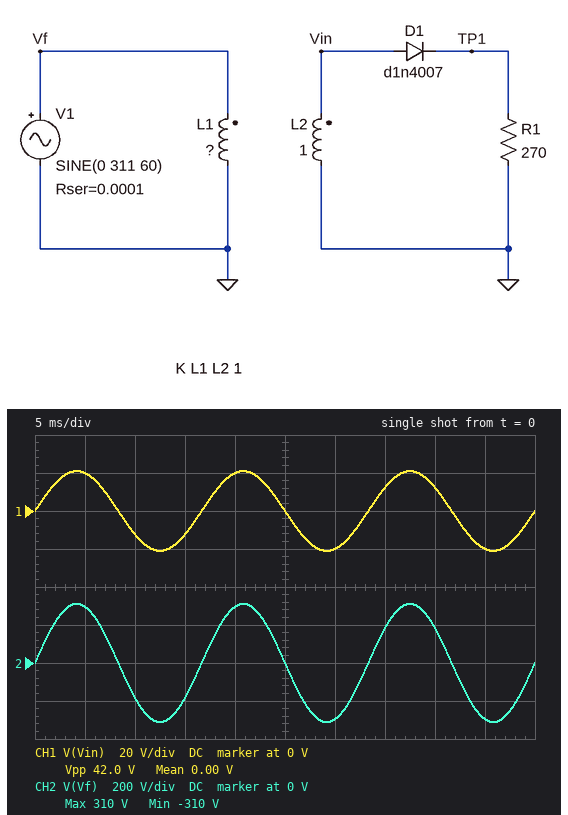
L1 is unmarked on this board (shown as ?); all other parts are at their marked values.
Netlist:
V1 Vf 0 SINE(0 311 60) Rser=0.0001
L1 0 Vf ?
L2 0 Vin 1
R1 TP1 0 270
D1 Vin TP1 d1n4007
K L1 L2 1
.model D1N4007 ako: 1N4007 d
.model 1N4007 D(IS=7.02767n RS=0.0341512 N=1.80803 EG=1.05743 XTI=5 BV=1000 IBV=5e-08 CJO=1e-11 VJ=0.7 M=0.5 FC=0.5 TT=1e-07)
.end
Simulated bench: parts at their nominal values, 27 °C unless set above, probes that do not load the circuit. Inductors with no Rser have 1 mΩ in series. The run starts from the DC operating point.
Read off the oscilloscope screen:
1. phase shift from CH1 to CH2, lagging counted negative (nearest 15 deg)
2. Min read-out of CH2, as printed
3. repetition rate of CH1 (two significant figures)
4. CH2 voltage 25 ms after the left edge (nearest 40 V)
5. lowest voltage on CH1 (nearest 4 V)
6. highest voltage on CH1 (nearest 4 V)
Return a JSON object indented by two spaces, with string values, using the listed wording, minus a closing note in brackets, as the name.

{
  "phase shift from CH1 to CH2, lagging counted negative": "0 deg",
  "Min read-out of CH2, as printed": "-310 V",
  "repetition rate of CH1": "60 Hz",
  "CH2 voltage 25 ms after the left edge": "0 V",
  "lowest voltage on CH1": "-20 V",
  "highest voltage on CH1": "20 V"
}
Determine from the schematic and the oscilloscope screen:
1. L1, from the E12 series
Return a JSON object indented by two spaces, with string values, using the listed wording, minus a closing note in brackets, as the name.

{
  "L1, from the E12 series": "220 H"
}
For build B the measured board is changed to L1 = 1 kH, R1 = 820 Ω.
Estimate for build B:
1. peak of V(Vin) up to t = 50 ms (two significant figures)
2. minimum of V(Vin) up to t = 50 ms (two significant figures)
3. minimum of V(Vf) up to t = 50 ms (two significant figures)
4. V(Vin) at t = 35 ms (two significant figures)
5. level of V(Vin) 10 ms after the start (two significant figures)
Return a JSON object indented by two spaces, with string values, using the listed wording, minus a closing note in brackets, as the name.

{
  "peak of V(Vin) up to t = 50 ms": "9.8 V",
  "minimum of V(Vin) up to t = 50 ms": "-9.8 V",
  "minimum of V(Vf) up to t = 50 ms": "-310 V",
  "V(Vin) at t = 35 ms": "5.8 V",
  "level of V(Vin) 10 ms after the start": "-5.8 V"
}
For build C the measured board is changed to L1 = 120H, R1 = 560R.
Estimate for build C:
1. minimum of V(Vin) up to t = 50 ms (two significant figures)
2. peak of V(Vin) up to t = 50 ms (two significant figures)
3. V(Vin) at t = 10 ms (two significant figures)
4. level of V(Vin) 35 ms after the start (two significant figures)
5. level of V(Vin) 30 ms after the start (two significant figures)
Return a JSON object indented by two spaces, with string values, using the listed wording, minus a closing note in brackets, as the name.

{
  "minimum of V(Vin) up to t = 50 ms": "-28 V",
  "peak of V(Vin) up to t = 50 ms": "28 V",
  "V(Vin) at t = 10 ms": "-17 V",
  "level of V(Vin) 35 ms after the start": "17 V",
  "level of V(Vin) 30 ms after the start": "-27 V"
}
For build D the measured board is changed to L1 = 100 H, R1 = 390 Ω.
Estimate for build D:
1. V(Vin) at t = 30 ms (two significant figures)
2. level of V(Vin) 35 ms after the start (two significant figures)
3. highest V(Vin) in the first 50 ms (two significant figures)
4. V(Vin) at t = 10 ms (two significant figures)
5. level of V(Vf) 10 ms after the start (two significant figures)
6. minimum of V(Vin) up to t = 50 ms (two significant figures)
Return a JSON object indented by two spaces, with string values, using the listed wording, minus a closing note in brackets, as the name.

{
  "V(Vin) at t = 30 ms": "-30 V",
  "level of V(Vin) 35 ms after the start": "18 V",
  "highest V(Vin) in the first 50 ms": "31 V",
  "V(Vin) at t = 10 ms": "-18 V",
  "level of V(Vf) 10 ms after the start": "-180 V",
  "minimum of V(Vin) up to t = 50 ms": "-31 V"
}
